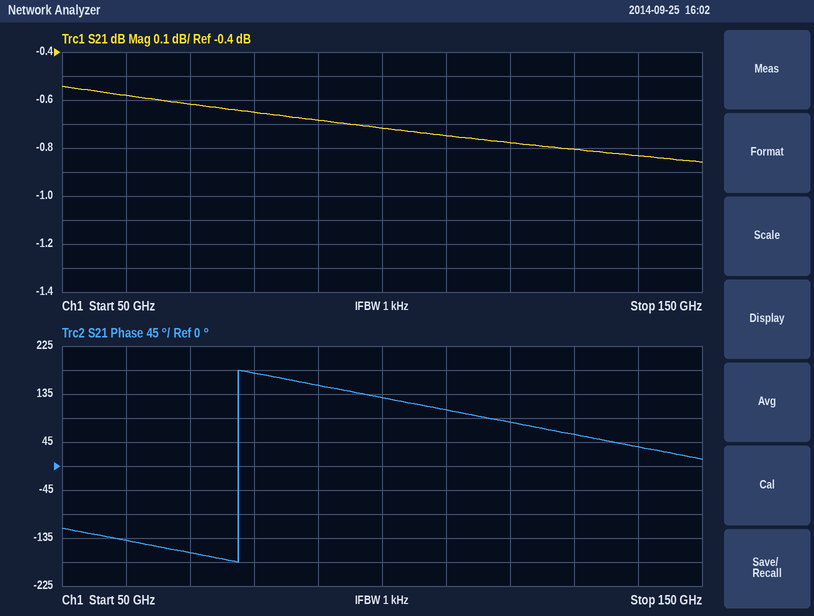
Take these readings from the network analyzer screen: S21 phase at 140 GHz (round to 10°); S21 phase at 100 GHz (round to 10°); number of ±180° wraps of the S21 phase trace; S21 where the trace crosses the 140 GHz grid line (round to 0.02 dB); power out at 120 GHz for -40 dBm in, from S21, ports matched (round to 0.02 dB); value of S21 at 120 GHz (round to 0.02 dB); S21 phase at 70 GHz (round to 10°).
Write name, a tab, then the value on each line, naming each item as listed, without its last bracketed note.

S21 phase at 140 GHz	40°
S21 phase at 100 GHz	130°
number of ±180° wraps of the S21 phase trace	1
S21 where the trace crosses the 140 GHz grid line	-0.84 dB
power out at 120 GHz for -40 dBm in, from S21, ports matched	-40.78 dBm
value of S21 at 120 GHz	-0.78 dB
S21 phase at 70 GHz	-160°
